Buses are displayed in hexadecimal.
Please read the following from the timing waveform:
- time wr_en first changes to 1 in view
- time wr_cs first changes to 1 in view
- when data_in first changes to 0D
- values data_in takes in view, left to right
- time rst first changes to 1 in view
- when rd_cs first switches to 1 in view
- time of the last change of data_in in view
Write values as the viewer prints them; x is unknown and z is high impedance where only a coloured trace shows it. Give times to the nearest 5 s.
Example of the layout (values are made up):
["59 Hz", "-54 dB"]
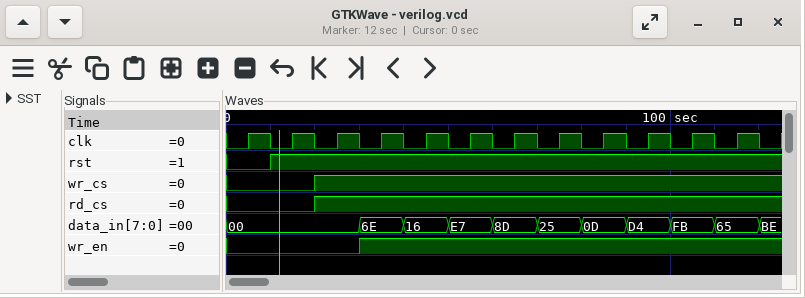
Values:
["30 s", "20 s", "80 s", "00, 6E, 16, E7, 8D, 25, 0D, D4, FB, 65, BE", "10 s", "20 s", "120 s"]
